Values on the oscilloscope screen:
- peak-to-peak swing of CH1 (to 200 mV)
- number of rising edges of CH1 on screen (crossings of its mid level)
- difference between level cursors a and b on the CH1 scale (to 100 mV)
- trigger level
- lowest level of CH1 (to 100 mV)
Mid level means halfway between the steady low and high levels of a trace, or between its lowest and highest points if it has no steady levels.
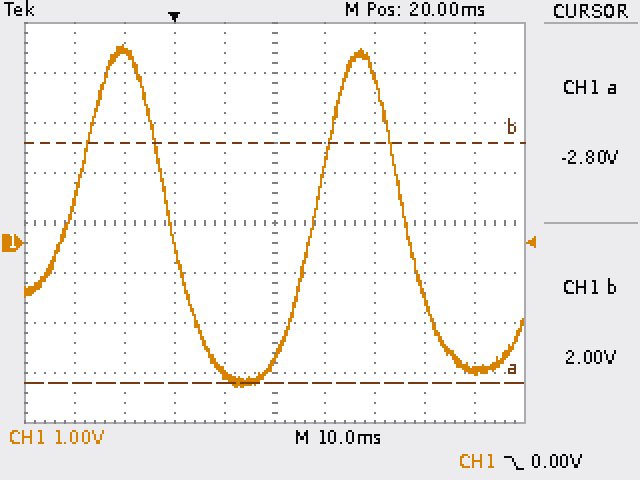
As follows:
6.8 V
2
4.8 V
0.00 V
-2.9 V
